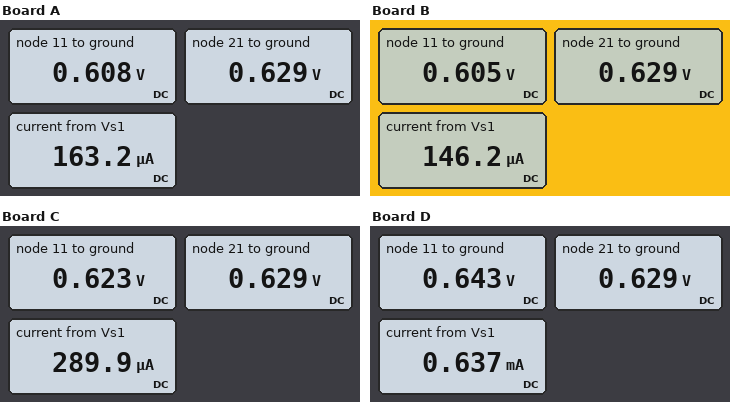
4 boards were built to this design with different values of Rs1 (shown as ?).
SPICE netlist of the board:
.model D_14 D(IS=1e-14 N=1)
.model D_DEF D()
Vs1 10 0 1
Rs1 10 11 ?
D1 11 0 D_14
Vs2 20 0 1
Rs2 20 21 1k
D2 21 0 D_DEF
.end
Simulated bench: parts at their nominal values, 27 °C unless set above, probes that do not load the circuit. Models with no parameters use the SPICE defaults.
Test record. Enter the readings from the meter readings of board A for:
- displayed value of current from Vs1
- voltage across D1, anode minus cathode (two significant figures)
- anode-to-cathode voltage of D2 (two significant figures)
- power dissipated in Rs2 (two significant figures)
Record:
163.2 µA
610 mV
630 mV
140 µW
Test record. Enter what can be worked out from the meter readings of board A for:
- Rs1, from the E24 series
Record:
2.4 kΩ
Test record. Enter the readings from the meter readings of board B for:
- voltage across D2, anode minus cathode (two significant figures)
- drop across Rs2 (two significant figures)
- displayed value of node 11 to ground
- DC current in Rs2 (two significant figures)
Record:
630 mV
370 mV
0.605 V
370 µA
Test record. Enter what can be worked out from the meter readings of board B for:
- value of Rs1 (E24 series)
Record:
2.7 kΩ
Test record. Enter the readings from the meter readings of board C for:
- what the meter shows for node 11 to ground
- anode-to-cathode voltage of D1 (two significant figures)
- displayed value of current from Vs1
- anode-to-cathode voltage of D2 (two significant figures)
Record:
0.623 V
620 mV
289.9 µA
630 mV
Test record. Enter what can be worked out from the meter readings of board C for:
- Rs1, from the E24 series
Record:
1.3 kΩ
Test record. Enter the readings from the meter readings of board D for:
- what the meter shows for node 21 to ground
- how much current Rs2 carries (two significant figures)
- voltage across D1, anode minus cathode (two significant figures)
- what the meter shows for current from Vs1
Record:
0.629 V
370 µA
640 mV
0.637 mA
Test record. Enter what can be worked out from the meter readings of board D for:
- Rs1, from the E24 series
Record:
560 Ω
